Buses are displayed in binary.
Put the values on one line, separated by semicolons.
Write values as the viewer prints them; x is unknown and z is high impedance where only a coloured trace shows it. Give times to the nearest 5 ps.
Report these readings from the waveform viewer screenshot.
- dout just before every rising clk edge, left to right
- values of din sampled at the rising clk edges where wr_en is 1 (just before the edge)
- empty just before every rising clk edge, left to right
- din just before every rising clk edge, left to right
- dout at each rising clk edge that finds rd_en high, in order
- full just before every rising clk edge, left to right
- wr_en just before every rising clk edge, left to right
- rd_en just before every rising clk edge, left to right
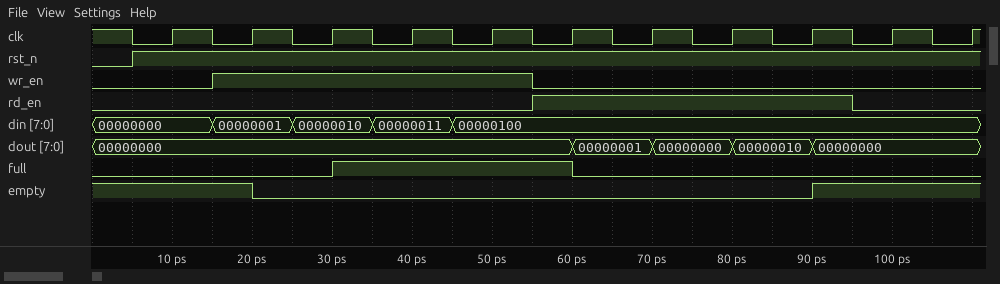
00000000, 00000000, 00000000, 00000000, 00000000, 00000000, 00000001, 00000000, 00000010, 00000000, 00000000; 00000001, 00000010, 00000011, 00000100; 1 1 0 0 0 0 0 0 0 1 1; 00000000, 00000001, 00000010, 00000011, 00000100, 00000100, 00000100, 00000100, 00000100, 00000100, 00000100; 00000000, 00000001, 00000000, 00000010; 0 0 0 1 1 1 0 0 0 0 0; 0 1 1 1 1 0 0 0 0 0 0; 0 0 0 0 0 1 1 1 1 0 0
